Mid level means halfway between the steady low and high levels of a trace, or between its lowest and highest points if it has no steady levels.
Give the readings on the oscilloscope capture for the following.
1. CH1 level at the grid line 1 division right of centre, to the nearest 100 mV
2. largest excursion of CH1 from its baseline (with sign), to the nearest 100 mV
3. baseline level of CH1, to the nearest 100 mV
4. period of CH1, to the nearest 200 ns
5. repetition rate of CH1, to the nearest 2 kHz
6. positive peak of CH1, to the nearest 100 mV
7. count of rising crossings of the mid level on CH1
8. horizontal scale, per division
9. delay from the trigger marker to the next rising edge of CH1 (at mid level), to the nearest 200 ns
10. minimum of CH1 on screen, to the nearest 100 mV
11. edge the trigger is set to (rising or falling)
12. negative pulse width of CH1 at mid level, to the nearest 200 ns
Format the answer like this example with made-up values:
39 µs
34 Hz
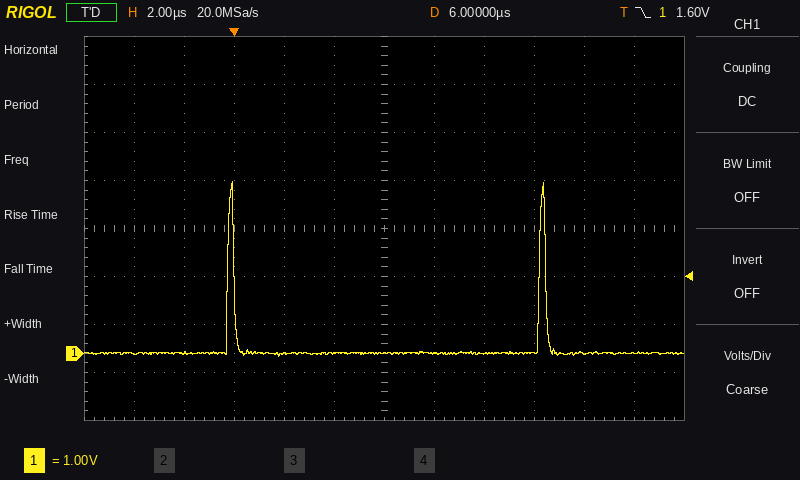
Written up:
0.0 V
+3.6 V
0.0 V
12.4 µs
80 kHz
3.6 V
2
2 µs
12.2 µs
-100 mV
falling
12.2 µs
